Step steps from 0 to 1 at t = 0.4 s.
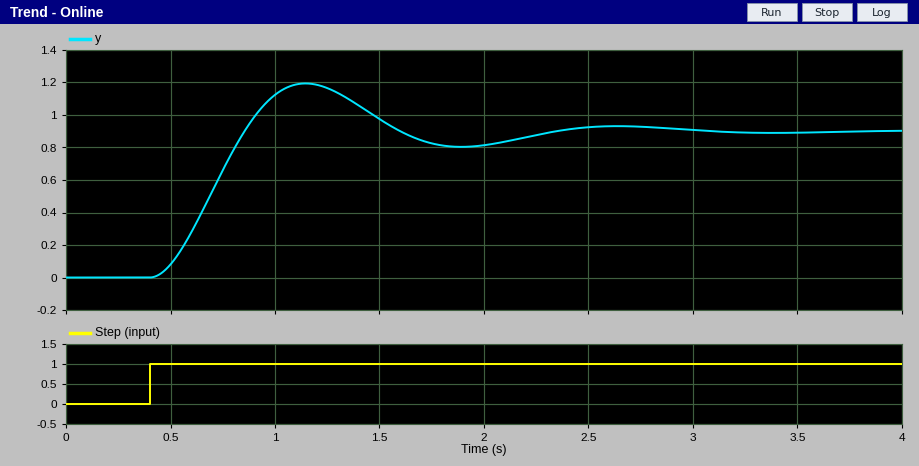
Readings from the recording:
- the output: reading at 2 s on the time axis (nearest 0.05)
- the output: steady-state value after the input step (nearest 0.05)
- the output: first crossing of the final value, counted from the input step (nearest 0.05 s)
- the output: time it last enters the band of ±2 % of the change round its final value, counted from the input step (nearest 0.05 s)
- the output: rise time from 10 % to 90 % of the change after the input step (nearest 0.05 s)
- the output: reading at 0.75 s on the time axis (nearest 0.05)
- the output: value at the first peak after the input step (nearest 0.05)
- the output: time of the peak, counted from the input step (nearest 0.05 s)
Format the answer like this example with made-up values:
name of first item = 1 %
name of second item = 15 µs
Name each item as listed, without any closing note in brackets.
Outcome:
the output: reading at 2 s on the time axis = 0.80
the output: steady-state value after the input step = 0.90
the output: first crossing of the final value, counted from the input step = 0.45 s
the output: time it last enters the band of ±2 % of the change round its final value, counted from the input step = 2.50 s
the output: rise time from 10 % to 90 % of the change after the input step = 0.30 s
the output: reading at 0.75 s on the time axis = 0.65
the output: value at the first peak after the input step = 1.20
the output: time of the peak, counted from the input step = 0.75 s
